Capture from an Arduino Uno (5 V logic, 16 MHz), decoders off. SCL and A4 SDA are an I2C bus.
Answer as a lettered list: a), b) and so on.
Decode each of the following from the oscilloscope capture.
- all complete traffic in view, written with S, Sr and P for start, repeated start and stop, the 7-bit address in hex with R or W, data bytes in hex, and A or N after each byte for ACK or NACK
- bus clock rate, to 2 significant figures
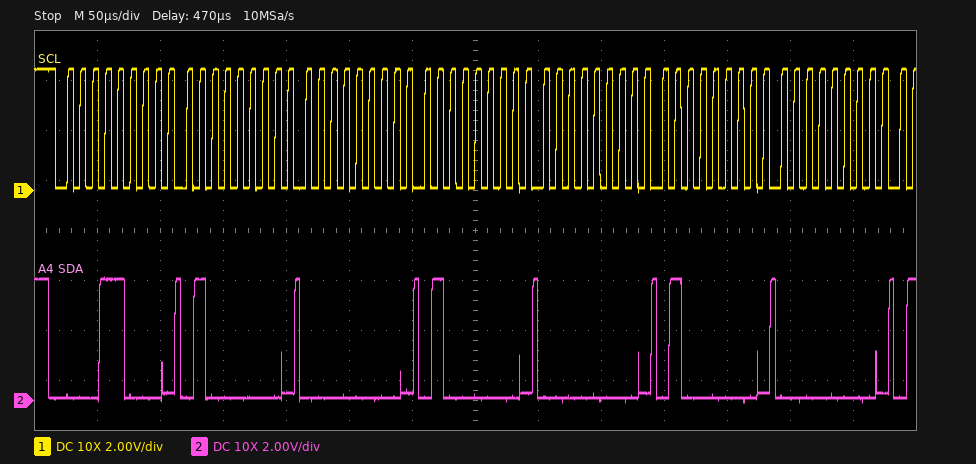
a) S 0CW A 40 A 00 A 40 A 00 A 40 A 00 A
b) 100 kHz
